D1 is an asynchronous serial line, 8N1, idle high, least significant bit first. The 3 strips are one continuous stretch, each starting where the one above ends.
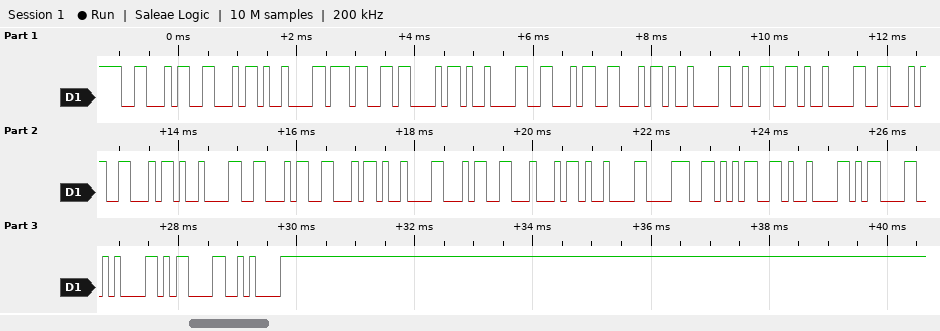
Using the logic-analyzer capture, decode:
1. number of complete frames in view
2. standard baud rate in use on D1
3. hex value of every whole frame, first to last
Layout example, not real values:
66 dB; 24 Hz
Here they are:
27; 9600 baud; 46 46 09 37 43 09 46 46 09 32 09 46 46 09 46 46 09 34 44 09 38 35 09 0D 0A 0D 0A
